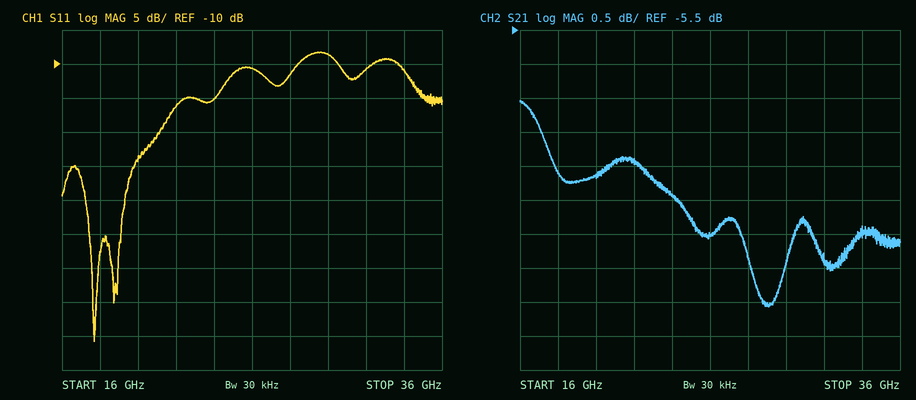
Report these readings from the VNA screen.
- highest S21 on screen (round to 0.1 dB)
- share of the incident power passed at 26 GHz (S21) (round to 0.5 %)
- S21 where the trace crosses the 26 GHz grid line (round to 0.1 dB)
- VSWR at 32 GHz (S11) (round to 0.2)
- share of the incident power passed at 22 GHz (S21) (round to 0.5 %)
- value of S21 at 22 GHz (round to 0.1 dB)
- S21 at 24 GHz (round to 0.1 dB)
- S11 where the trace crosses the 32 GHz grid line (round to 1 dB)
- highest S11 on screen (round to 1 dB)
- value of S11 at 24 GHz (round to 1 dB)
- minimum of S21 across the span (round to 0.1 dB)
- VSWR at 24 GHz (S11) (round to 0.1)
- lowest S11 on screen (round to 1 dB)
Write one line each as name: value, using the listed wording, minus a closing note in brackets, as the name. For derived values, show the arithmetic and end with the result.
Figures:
highest S21 on screen: -6.5 dB
share of the incident power passed at 26 GHz (S21): 10^(-8.5/10) ≈ 14.1 %, so 14.0 % to the nearest 0.5 %
S21 where the trace crosses the 26 GHz grid line: -8.5 dB
VSWR at 32 GHz (S11): |Γ| = 10^(-11/20) = 0.2818; VSWR = (1 + 0.2818)/(1 − 0.2818) ≈ 1.8
share of the incident power passed at 22 GHz (S21): 10^(-7.4/10) ≈ 18.2 %, so 18.0 % to the nearest 0.5 %
value of S21 at 22 GHz: -7.4 dB
S21 at 24 GHz: -7.9 dB
S11 where the trace crosses the 32 GHz grid line: -11 dB
highest S11 on screen: -8 dB
value of S11 at 24 GHz: -15 dB
minimum of S21 across the span: -9.6 dB
VSWR at 24 GHz (S11): |Γ| = 10^(-15/20) = 0.1778; VSWR = (1 + 0.1778)/(1 − 0.1778) ≈ 1.4
lowest S11 on screen: -51 dB
